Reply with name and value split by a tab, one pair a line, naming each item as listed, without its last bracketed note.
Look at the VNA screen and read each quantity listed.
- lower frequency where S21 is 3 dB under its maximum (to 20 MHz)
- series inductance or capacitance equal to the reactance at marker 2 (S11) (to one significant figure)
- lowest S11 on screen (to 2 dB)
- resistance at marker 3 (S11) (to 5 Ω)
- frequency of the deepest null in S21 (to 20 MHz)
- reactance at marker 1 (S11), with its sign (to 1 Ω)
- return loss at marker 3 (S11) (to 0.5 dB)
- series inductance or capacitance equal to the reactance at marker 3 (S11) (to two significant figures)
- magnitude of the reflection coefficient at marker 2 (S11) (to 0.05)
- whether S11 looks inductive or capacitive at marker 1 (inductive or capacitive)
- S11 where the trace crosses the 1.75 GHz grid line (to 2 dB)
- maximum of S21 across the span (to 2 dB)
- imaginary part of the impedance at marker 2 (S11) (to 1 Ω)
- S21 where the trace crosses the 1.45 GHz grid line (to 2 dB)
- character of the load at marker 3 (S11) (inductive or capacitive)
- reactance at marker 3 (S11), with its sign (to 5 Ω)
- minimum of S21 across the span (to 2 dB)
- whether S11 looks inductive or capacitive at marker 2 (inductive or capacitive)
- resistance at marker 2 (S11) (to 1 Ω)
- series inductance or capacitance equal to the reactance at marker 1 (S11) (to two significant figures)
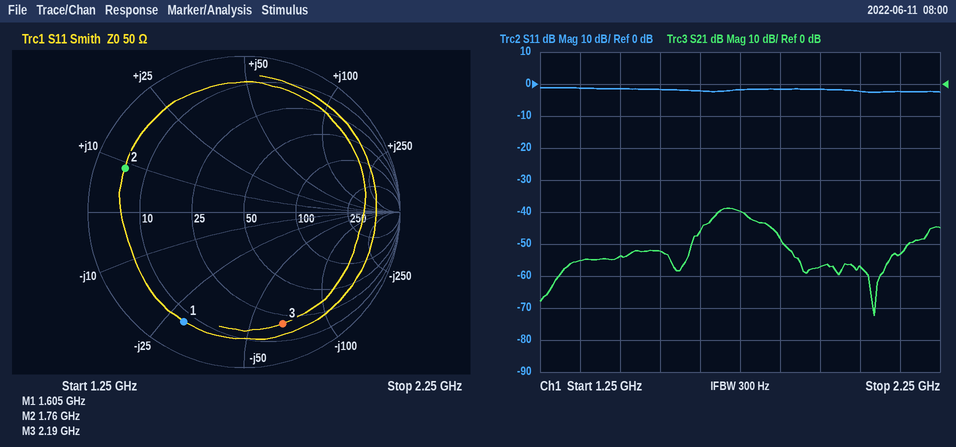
lower frequency where S21 is 3 dB under its maximum	1.68 GHz
series inductance or capacitance equal to the reactance at marker 2 (S11)	800 pH
lowest S11 on screen	-2 dB
resistance at marker 3 (S11)	20 Ω
frequency of the deepest null in S21	2.08 GHz
reactance at marker 1 (S11), with its sign	-29 Ω
return loss at marker 3 (S11)	2.5 dB
series inductance or capacitance equal to the reactance at marker 3 (S11)	1.1 pF
magnitude of the reflection coefficient at marker 2 (S11)	0.80
whether S11 looks inductive or capacitive at marker 1	capacitive
S11 where the trace crosses the 1.75 GHz grid line	-2 dB
maximum of S21 across the span	-38 dB
imaginary part of the impedance at marker 2 (S11)	+9 Ω
S21 where the trace crosses the 1.45 GHz grid line	-54 dB
character of the load at marker 3 (S11)	capacitive
reactance at marker 3 (S11), with its sign	-65 Ω
minimum of S21 across the span	-72 dB
whether S11 looks inductive or capacitive at marker 2	inductive
resistance at marker 2 (S11)	5 Ω
series inductance or capacitance equal to the reactance at marker 1 (S11)	3.4 pF
